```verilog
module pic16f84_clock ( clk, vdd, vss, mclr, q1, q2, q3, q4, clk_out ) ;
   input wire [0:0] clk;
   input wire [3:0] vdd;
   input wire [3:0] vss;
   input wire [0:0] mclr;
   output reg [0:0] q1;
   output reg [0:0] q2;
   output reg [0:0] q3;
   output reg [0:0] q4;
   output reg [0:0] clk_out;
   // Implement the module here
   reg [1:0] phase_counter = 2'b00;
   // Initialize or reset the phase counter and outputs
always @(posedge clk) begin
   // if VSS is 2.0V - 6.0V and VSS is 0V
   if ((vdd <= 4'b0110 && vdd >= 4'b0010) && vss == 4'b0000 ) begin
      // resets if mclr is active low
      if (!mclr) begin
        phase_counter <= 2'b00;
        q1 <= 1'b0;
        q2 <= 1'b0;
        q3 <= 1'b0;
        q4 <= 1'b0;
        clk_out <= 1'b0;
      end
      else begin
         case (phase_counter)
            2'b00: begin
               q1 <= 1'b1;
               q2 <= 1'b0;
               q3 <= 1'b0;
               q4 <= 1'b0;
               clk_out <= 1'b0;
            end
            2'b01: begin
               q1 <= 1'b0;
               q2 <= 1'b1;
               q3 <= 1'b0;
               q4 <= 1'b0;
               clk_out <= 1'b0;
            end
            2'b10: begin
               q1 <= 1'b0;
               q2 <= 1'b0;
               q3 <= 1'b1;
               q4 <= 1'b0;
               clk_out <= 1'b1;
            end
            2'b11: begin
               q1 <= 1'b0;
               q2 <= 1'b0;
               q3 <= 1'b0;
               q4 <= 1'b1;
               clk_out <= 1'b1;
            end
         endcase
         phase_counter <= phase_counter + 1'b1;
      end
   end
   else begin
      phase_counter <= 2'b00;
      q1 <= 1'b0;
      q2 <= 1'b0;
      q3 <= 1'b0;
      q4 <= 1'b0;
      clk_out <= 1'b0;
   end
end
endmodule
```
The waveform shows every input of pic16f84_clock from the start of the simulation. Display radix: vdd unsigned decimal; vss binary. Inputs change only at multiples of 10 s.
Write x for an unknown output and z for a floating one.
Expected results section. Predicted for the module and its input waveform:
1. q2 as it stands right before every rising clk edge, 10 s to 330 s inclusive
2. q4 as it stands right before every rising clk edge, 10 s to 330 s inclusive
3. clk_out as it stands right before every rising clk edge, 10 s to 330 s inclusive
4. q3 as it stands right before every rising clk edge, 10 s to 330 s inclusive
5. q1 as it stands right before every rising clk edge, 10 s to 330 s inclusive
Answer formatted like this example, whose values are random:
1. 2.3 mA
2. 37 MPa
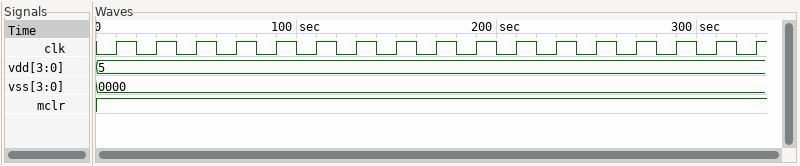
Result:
1. x 0 1 0 0 0 1 0 0 0 1 0 0 0 1 0 0
2. x 0 0 0 1 0 0 0 1 0 0 0 1 0 0 0 1
3. x 0 0 1 1 0 0 1 1 0 0 1 1 0 0 1 1
4. x 0 0 1 0 0 0 1 0 0 0 1 0 0 0 1 0
5. x 1 0 0 0 1 0 0 0 1 0 0 0 1 0 0 0
